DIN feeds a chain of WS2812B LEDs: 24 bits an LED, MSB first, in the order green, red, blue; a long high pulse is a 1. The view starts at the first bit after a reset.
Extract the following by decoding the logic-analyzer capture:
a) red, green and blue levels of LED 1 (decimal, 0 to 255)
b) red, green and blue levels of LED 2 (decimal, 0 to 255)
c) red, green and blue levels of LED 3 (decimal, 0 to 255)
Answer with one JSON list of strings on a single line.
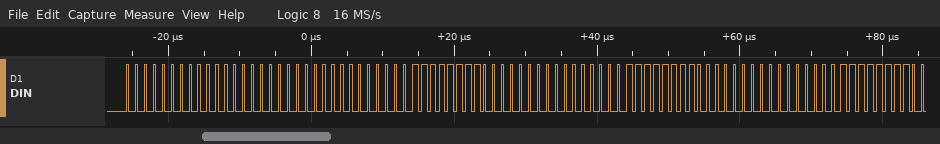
["0, 0, 0", "255, 0, 0", "255, 0, 0"]
